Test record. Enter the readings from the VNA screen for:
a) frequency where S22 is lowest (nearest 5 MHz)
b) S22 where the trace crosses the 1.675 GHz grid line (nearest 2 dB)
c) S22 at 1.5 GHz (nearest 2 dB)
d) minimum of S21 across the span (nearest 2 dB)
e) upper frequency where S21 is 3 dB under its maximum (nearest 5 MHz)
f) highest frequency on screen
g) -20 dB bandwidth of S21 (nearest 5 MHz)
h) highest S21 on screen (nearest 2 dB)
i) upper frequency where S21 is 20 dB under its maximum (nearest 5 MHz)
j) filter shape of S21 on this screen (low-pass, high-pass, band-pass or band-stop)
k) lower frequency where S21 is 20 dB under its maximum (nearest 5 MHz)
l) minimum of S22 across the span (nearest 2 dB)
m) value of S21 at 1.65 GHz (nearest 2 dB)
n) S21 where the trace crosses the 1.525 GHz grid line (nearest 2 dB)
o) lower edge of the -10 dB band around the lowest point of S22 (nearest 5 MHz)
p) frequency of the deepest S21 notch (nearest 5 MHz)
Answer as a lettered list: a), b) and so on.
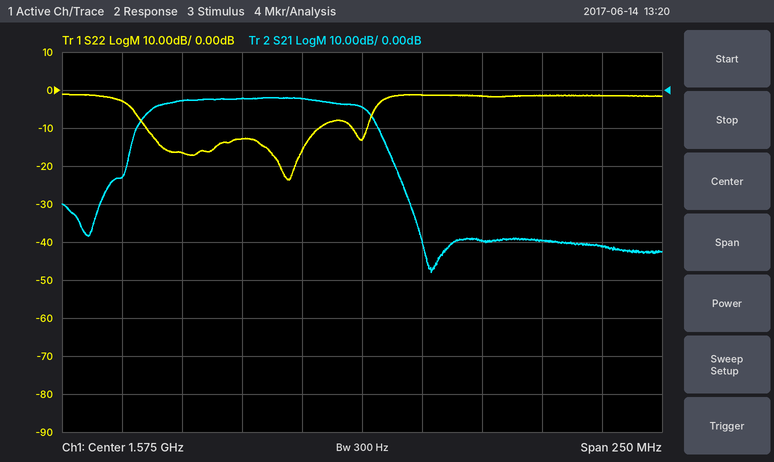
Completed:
a) 1.545 GHz
b) -2 dB
c) -16 dB
d) -48 dB
e) 1.575 GHz
f) 1.7 GHz
g) 115 MHz
h) -2 dB
i) 1.590 GHz
j) band-pass
k) 1.475 GHz
l) -24 dB
m) -40 dB
n) -2 dB
o) 1.485 GHz
p) 1.605 GHz
